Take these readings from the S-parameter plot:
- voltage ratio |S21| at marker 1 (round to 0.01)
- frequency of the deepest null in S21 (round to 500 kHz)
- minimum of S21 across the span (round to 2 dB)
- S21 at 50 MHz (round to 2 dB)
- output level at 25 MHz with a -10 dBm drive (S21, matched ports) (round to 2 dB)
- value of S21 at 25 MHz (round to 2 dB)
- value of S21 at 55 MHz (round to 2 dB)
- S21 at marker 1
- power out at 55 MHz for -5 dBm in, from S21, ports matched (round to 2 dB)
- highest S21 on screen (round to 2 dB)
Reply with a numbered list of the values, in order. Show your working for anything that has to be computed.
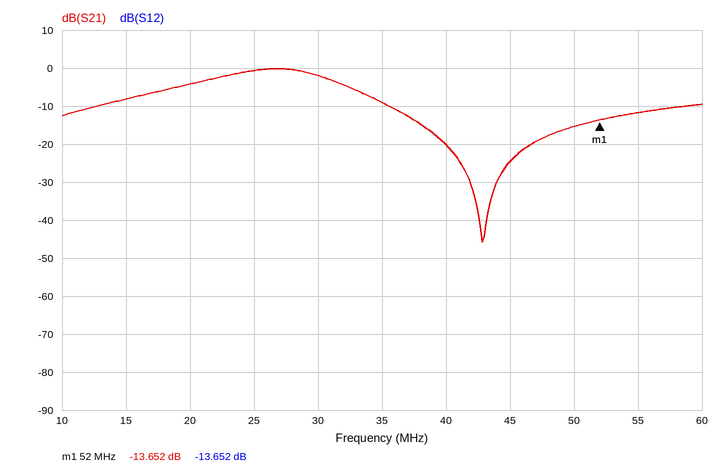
1. 10^(-13.652/20) ≈ 0.21
2. 43.0 MHz
3. -46 dB
4. -16 dB
5. -10 dBm + (0 dB) = -10 dBm
6. 0 dB
7. -12 dB
8. -13.652 dB
9. -5 dBm + (-12 dB) = -16 dBm
10. 0 dB
